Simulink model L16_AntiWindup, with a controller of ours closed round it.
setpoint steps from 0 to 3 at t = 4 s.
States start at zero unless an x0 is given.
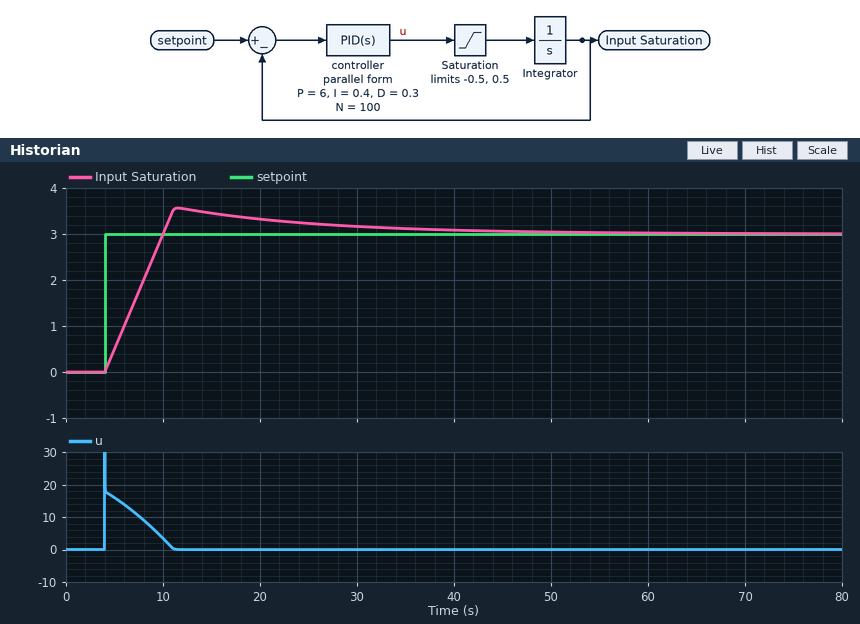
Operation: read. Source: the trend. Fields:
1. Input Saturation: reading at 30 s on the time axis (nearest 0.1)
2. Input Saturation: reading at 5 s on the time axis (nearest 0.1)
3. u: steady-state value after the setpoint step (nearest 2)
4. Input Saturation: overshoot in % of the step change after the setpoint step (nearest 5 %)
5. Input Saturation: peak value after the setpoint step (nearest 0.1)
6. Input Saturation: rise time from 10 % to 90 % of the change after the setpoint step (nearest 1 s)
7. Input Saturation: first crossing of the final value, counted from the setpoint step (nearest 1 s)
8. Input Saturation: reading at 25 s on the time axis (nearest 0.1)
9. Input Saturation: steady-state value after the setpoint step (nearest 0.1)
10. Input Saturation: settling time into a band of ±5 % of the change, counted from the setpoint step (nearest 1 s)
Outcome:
3.2
0.5
0
20 %
3.6
5 s
6 s
3.2
3.0
27 s
